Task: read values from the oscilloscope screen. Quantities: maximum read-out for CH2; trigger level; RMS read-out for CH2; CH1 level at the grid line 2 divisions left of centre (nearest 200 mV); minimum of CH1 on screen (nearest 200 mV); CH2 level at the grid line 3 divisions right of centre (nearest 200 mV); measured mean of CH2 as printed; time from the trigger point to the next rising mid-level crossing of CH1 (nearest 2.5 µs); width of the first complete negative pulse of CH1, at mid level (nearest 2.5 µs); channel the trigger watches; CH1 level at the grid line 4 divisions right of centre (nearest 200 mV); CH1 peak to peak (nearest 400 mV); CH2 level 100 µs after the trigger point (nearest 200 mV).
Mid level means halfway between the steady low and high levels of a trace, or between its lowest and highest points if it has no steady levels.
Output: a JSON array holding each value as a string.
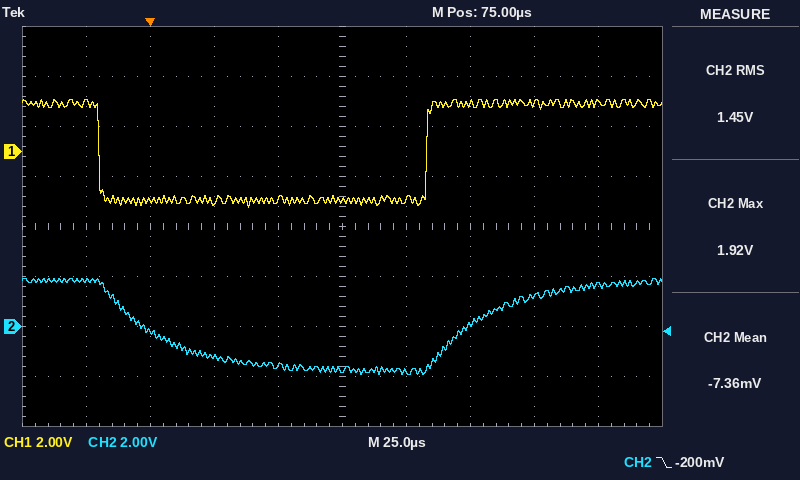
["1.92 V", "-200 mV", "1.45 V", "-2.0 V", "-2.2 V", "1.2 V", "-7.36 mV", "107.5 µs", "127.5 µs", "CH2", "2.0 V", "4.4 V", "-1.8 V"]
